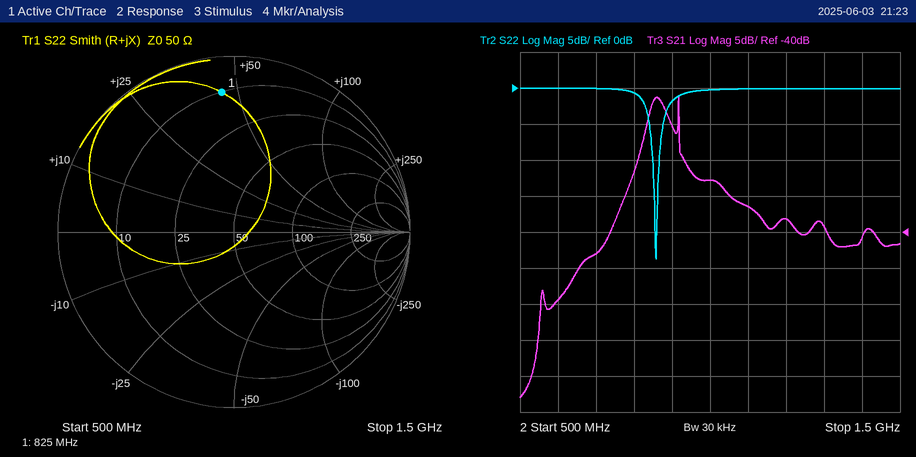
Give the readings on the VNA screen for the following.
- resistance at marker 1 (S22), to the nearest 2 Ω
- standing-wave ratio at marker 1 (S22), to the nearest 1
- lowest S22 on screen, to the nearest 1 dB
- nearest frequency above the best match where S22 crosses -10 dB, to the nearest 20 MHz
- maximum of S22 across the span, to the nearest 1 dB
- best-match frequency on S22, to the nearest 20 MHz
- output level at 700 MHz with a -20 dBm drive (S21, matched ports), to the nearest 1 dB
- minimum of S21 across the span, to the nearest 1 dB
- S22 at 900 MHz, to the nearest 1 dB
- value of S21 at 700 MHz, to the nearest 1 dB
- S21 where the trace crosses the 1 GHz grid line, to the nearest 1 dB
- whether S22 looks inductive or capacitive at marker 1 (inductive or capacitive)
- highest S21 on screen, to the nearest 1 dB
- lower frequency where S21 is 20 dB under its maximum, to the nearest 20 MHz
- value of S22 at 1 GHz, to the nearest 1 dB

10 Ω
9
-24 dB
860 MHz
0 dB
860 MHz
-63 dBm
-63 dB
-2 dB
-43 dB
-33 dB
inductive
-21 dB
720 MHz
0 dB
